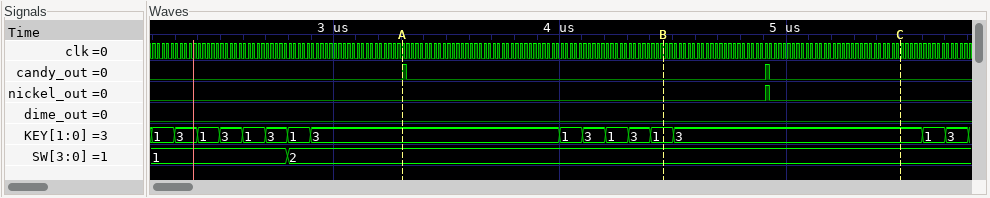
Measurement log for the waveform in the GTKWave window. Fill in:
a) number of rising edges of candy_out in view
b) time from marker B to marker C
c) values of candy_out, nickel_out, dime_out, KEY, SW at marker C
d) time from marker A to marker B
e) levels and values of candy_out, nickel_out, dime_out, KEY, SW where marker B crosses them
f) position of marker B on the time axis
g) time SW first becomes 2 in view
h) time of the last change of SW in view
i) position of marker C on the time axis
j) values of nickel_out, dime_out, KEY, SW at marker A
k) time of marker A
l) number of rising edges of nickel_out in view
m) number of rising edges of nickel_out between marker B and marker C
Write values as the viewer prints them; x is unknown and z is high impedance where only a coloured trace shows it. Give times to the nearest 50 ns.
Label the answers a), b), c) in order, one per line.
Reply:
a) 2
b) 1050 ns
c) candy_out=0, nickel_out=0, dime_out=0, KEY=3, SW=2
d) 1150 ns
e) candy_out=0, nickel_out=0, dime_out=0, KEY=1, SW=2
f) 4450 ns
g) 2800 ns
h) 2800 ns
i) 5500 ns
j) nickel_out=0, dime_out=0, KEY=3, SW=2
k) 3300 ns
l) 1
m) 1
